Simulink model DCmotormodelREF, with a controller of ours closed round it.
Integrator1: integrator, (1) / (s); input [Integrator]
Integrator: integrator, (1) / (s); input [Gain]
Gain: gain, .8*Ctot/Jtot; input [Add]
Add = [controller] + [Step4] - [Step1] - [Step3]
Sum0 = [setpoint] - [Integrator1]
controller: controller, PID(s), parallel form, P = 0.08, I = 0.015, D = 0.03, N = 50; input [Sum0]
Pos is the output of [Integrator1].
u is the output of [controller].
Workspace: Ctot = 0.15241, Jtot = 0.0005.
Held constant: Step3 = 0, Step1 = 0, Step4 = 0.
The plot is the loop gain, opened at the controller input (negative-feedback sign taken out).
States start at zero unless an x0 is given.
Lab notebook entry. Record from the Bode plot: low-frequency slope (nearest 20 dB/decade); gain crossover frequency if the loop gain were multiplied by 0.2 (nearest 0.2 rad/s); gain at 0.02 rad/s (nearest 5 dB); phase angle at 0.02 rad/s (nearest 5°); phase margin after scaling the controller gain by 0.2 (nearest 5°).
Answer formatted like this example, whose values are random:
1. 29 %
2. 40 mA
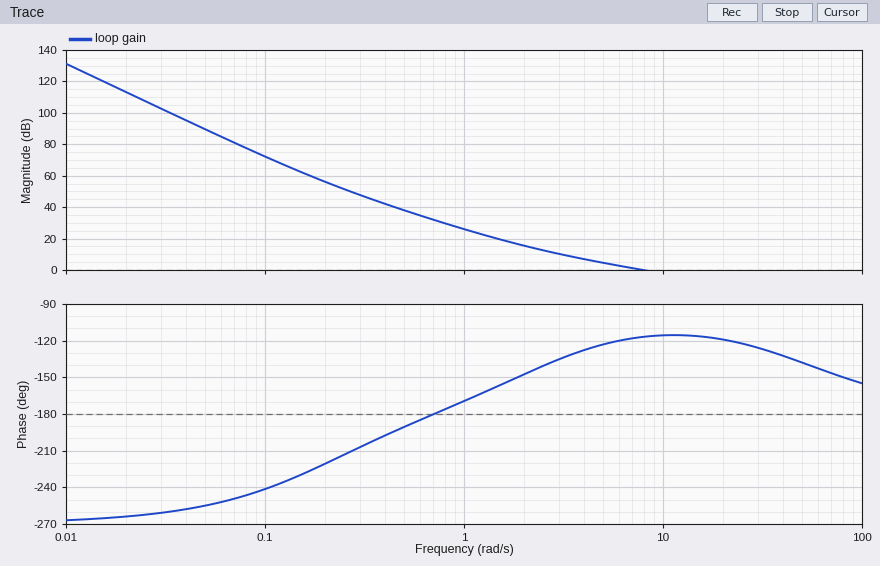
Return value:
1. -60 dB/decade
2. 2.2 rad/s
3. 115 dB
4. -265°
5. 35°
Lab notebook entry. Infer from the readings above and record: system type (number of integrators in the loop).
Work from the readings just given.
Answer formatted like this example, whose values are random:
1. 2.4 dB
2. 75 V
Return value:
1. 3
